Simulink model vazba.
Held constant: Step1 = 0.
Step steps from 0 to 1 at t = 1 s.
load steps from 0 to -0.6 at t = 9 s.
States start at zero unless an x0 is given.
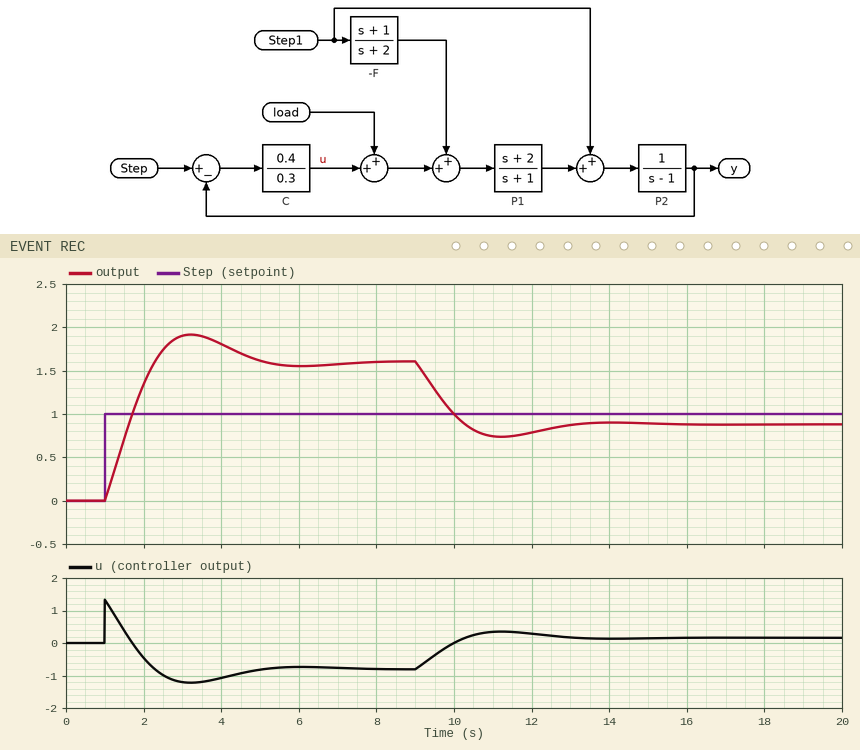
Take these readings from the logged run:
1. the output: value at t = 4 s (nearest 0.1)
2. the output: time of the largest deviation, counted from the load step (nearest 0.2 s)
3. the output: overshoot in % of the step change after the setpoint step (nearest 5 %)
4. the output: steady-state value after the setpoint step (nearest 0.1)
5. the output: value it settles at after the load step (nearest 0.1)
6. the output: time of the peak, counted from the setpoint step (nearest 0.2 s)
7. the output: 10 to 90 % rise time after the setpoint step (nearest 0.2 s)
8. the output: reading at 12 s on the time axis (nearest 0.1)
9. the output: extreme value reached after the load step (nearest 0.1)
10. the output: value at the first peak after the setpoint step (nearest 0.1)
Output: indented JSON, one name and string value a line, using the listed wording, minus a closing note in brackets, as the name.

{
  "the output: value at t = 4 s": "1.8",
  "the output: time of the largest deviation, counted from the load step": "2.2 s",
  "the output: overshoot in % of the step change after the setpoint step": "20 %",
  "the output: steady-state value after the setpoint step": "1.6",
  "the output: value it settles at after the load step": "0.9",
  "the output: time of the peak, counted from the setpoint step": "2.2 s",
  "the output: 10 to 90 % rise time after the setpoint step": "1.0 s",
  "the output: reading at 12 s on the time axis": "0.8",
  "the output: extreme value reached after the load step": "0.7",
  "the output: value at the first peak after the setpoint step": "1.9"
}
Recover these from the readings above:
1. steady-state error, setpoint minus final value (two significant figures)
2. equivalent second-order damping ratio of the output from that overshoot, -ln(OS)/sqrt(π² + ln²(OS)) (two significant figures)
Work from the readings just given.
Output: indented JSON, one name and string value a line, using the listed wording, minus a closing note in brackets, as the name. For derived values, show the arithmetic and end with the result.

{
  "steady-state error, setpoint minus final value": "1 - 1.6 = -0.60",
  "equivalent second-order damping ratio of the output from that overshoot, -ln(OS)/sqrt(π² + ln²(OS))": "ln(0.2) = -1.609; 1.609 / sqrt(9.870 + 2.590) = 0.46"
}
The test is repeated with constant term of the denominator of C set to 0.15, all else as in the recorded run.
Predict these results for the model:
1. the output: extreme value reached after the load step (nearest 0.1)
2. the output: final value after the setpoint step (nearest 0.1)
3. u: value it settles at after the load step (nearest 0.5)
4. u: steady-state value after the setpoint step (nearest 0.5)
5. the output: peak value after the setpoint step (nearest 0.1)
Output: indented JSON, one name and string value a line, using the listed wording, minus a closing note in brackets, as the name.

{
  "the output: extreme value reached after the load step": "0.9",
  "the output: final value after the setpoint step": "1.2",
  "u: value it settles at after the load step": "0.0",
  "u: steady-state value after the setpoint step": "-0.5",
  "the output: peak value after the setpoint step": "1.4"
}
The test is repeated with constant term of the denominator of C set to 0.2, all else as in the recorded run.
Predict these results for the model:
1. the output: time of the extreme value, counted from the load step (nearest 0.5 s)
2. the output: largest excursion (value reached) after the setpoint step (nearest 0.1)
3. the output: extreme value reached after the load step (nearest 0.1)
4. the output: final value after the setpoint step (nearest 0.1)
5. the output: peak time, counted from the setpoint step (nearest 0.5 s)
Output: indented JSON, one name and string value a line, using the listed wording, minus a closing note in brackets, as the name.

{
  "the output: time of the extreme value, counted from the load step": "1.5 s",
  "the output: largest excursion (value reached) after the setpoint step": "1.6",
  "the output: extreme value reached after the load step": "0.9",
  "the output: final value after the setpoint step": "1.3",
  "the output: peak time, counted from the setpoint step": "1.5 s"
}
